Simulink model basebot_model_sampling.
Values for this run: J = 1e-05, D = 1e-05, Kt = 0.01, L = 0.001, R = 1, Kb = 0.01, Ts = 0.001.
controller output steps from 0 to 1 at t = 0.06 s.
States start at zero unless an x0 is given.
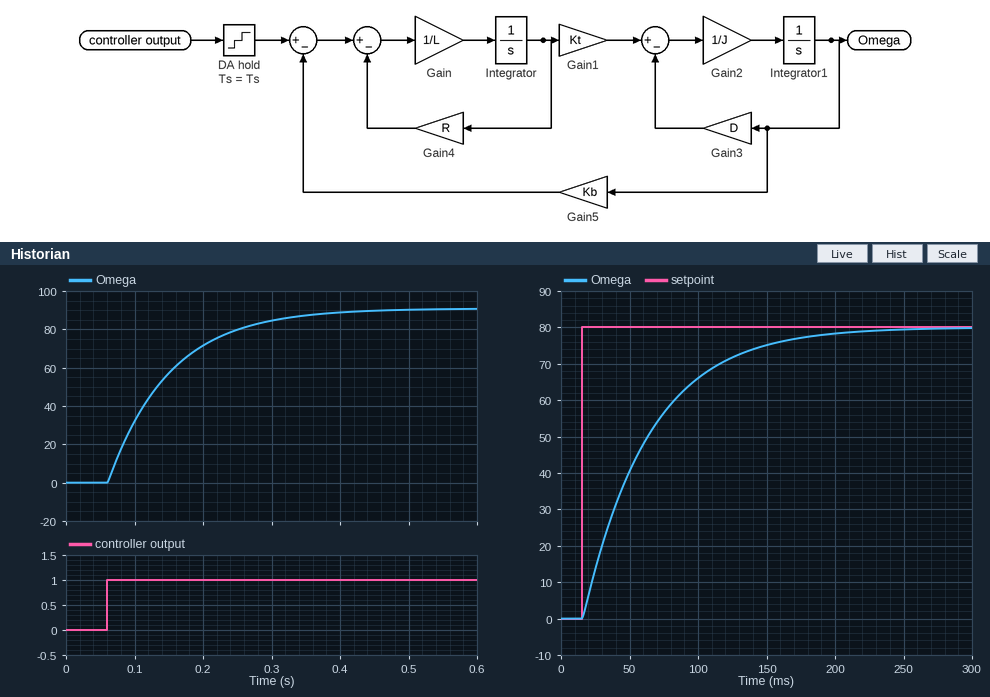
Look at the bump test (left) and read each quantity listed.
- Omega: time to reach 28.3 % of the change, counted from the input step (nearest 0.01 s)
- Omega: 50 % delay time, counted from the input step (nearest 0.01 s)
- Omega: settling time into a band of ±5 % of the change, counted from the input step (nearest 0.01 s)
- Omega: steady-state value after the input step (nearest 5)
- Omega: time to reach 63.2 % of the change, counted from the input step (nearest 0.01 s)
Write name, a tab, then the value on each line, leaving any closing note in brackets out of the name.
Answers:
Omega: time to reach 28.3 % of the change, counted from the input step	0.03 s
Omega: 50 % delay time, counted from the input step	0.06 s
Omega: settling time into a band of ±5 % of the change, counted from the input step	0.27 s
Omega: steady-state value after the input step	90
Omega: time to reach 63.2 % of the change, counted from the input step	0.09 s
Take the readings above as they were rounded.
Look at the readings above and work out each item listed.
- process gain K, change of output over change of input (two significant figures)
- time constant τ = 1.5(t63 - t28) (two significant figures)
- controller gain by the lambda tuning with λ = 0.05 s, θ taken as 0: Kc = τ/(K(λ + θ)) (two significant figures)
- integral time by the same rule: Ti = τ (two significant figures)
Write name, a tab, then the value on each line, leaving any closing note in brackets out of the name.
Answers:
process gain K, change of output over change of input	90
time constant τ = 1.5(t63 - t28)	0.090 s
controller gain by the lambda tuning with λ = 0.05 s, θ taken as 0: Kc = τ/(K(λ + θ))	0.020
integral time by the same rule: Ti = τ	0.090 s
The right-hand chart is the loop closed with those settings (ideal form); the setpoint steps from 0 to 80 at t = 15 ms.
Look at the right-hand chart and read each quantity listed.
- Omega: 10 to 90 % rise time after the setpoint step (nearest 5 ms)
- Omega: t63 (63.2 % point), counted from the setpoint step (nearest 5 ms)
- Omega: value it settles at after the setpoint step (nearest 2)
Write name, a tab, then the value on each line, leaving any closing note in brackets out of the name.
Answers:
Omega: 10 to 90 % rise time after the setpoint step	105 ms
Omega: t63 (63.2 % point), counted from the setpoint step	50 ms
Omega: value it settles at after the setpoint step	80
